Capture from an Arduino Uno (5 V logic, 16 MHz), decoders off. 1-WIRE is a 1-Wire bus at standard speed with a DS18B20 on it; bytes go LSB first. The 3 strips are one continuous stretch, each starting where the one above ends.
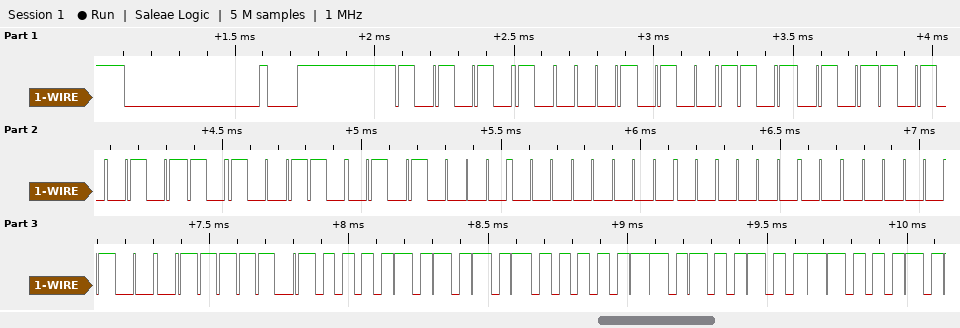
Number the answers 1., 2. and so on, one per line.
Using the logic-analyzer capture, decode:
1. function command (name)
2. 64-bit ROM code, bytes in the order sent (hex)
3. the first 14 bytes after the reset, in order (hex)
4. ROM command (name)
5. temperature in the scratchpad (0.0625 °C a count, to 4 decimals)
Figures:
1. Read Scratchpad
2. 28 AB A5 65 0A 00 00 20
3. 55 28 AB A5 65 0A 00 00 20 BE 50 05 4B 46
4. Match ROM
5. 85.0000 °C
